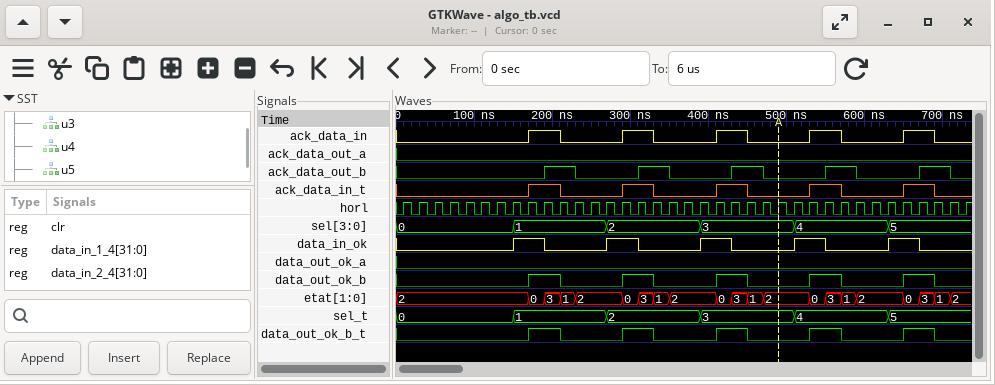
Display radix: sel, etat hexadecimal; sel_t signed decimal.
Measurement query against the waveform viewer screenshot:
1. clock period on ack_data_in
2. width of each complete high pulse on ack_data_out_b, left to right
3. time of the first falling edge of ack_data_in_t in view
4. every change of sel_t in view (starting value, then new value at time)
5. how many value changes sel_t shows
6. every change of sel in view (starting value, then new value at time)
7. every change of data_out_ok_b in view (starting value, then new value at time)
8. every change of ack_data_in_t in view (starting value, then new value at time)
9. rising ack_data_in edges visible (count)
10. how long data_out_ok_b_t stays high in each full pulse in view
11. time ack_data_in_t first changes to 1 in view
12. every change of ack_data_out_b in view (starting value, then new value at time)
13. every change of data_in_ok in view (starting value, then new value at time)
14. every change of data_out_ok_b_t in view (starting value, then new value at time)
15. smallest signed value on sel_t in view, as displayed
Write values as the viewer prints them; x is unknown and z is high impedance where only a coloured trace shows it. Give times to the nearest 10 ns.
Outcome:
120 ns
40 ns, 40 ns, 40 ns, 40 ns, 40 ns
210 ns
0, 1 at 150 ns, 2 at 270 ns, 3 at 390 ns, 4 at 510 ns, 5 at 630 ns
5
0, 1 at 150 ns, 2 at 270 ns, 3 at 390 ns, 4 at 510 ns, 5 at 630 ns
0, 1 at 170 ns, 0 at 210 ns, 1 at 290 ns, 0 at 330 ns, 1 at 410 ns, 0 at 450 ns, 1 at 530 ns, 0 at 570 ns, 1 at 650 ns, 0 at 690 ns
0, 1 at 170 ns, 0 at 210 ns, 1 at 290 ns, 0 at 330 ns, 1 at 410 ns, 0 at 450 ns, 1 at 530 ns, 0 at 570 ns, 1 at 650 ns, 0 at 690 ns
5
40 ns, 40 ns, 40 ns, 40 ns, 40 ns
170 ns
0, 1 at 190 ns, 0 at 230 ns, 1 at 310 ns, 0 at 350 ns, 1 at 430 ns, 0 at 470 ns, 1 at 550 ns, 0 at 590 ns, 1 at 670 ns, 0 at 710 ns
0, 1 at 150 ns, 0 at 190 ns, 1 at 270 ns, 0 at 310 ns, 1 at 390 ns, 0 at 430 ns, 1 at 510 ns, 0 at 550 ns, 1 at 630 ns, 0 at 670 ns
0, 1 at 170 ns, 0 at 210 ns, 1 at 290 ns, 0 at 330 ns, 1 at 410 ns, 0 at 450 ns, 1 at 530 ns, 0 at 570 ns, 1 at 650 ns, 0 at 690 ns
0
